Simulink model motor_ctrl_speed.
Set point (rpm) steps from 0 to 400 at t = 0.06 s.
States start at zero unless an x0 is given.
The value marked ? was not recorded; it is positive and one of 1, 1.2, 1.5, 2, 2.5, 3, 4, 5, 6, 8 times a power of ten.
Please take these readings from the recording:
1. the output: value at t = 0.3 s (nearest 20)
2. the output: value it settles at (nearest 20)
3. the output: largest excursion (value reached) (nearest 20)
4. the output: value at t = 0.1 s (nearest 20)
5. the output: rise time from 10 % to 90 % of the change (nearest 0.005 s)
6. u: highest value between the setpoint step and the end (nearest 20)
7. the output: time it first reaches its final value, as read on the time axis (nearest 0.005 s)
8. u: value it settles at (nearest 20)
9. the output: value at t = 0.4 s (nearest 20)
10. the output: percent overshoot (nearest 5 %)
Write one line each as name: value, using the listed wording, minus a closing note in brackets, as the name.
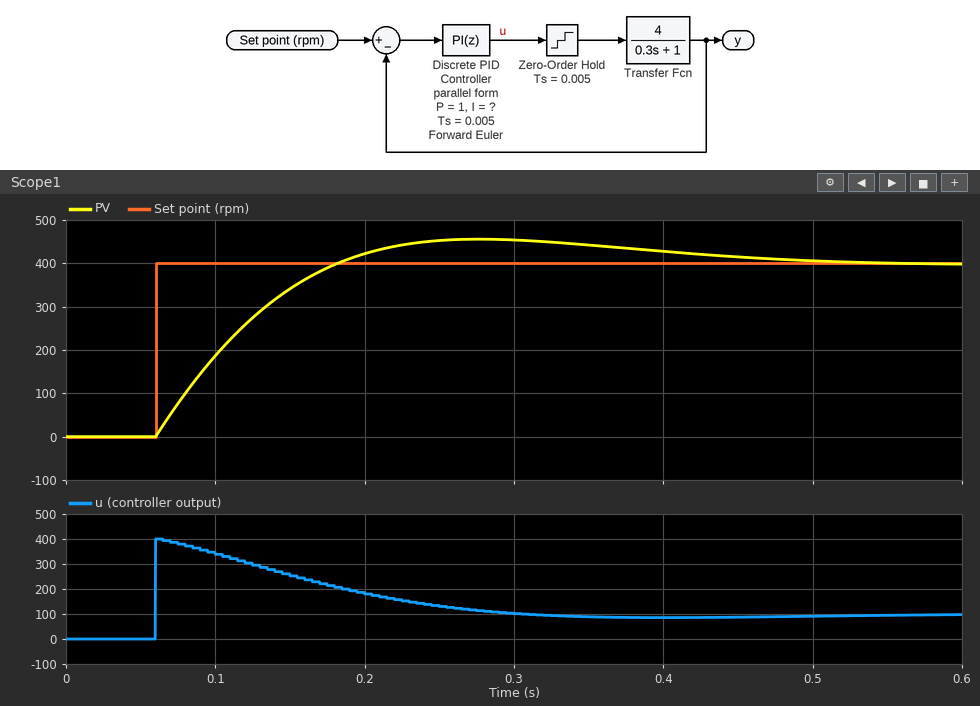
the output: value at t = 0.3 s: 460
the output: value it settles at: 400
the output: largest excursion (value reached): 460
the output: value at t = 0.1 s: 180
the output: rise time from 10 % to 90 % of the change: 0.090 s
u: highest value between the setpoint step and the end: 400
the output: time it first reaches its final value, as read on the time axis: 0.180 s
u: value it settles at: 100
the output: value at t = 0.4 s: 420
the output: percent overshoot: 15 %
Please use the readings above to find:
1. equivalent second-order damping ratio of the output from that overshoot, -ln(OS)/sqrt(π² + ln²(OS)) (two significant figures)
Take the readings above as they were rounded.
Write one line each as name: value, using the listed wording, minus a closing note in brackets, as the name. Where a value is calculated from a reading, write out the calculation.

equivalent second-order damping ratio of the output from that overshoot, -ln(OS)/sqrt(π² + ln²(OS)): ln(0.15) = -1.897; 1.897 / sqrt(9.870 + 3.599) = 0.52
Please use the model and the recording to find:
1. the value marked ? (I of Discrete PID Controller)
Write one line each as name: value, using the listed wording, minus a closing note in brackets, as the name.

the value marked ?: 10
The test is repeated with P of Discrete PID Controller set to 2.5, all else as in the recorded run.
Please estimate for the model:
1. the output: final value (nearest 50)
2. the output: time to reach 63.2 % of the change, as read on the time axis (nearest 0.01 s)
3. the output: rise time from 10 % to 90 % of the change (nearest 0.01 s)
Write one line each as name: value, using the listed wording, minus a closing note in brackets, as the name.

the output: final value: 400
the output: time to reach 63.2 % of the change, as read on the time axis: 0.09 s
the output: rise time from 10 % to 90 % of the change: 0.06 s
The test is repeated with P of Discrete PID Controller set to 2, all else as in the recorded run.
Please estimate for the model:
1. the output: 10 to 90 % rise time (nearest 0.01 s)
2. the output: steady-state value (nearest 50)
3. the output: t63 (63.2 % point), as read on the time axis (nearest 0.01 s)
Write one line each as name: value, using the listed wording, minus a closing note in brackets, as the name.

the output: 10 to 90 % rise time: 0.07 s
the output: steady-state value: 400
the output: t63 (63.2 % point), as read on the time axis: 0.09 s
